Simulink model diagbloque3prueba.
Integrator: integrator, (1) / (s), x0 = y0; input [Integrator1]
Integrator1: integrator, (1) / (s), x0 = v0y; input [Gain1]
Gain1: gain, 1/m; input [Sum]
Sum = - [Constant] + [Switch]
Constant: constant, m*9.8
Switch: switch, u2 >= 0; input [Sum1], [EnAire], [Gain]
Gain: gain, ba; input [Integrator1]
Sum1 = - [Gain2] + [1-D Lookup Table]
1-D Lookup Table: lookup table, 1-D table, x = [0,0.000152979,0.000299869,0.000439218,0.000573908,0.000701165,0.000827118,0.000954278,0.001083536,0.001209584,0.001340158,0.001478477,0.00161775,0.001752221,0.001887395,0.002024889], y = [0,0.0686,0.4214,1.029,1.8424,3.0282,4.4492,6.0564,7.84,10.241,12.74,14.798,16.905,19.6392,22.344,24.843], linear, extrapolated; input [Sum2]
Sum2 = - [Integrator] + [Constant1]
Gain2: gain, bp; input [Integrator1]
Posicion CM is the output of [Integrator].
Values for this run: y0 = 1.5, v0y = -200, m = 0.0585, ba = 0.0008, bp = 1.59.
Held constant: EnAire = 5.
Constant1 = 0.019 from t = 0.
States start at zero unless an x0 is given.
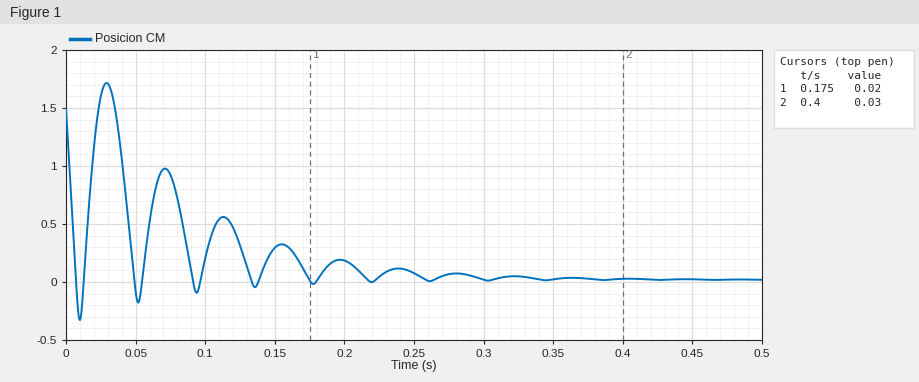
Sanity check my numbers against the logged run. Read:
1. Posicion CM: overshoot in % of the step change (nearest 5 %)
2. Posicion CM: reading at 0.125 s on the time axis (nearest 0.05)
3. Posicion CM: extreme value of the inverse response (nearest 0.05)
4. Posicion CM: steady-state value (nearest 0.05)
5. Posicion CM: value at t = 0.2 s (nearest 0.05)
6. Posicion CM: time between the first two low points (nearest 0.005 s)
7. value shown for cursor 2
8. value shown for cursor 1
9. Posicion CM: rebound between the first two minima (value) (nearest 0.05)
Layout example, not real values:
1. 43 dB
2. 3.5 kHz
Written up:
1. 25 %
2. 0.30
3. 1.70
4. 0.00
5. 0.20
6. 0.040 s
7. 0.03
8. 0.02
9. 1.70
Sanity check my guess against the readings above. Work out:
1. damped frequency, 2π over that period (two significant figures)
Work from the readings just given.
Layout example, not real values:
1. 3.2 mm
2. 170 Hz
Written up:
1. 160 rad/s
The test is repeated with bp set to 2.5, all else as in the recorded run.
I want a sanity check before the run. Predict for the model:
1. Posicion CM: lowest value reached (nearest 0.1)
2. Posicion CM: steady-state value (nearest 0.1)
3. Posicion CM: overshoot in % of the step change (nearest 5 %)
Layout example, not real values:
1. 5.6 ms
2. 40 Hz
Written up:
1. -0.3
2. 0.0
3. 20 %
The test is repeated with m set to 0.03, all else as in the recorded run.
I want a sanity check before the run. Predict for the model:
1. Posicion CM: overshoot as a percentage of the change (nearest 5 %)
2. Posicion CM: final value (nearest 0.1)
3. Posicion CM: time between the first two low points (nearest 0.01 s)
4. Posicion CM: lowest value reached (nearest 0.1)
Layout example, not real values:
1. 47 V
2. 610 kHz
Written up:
1. 15 %
2. 0.0
3. 0.03 s
4. -0.2
